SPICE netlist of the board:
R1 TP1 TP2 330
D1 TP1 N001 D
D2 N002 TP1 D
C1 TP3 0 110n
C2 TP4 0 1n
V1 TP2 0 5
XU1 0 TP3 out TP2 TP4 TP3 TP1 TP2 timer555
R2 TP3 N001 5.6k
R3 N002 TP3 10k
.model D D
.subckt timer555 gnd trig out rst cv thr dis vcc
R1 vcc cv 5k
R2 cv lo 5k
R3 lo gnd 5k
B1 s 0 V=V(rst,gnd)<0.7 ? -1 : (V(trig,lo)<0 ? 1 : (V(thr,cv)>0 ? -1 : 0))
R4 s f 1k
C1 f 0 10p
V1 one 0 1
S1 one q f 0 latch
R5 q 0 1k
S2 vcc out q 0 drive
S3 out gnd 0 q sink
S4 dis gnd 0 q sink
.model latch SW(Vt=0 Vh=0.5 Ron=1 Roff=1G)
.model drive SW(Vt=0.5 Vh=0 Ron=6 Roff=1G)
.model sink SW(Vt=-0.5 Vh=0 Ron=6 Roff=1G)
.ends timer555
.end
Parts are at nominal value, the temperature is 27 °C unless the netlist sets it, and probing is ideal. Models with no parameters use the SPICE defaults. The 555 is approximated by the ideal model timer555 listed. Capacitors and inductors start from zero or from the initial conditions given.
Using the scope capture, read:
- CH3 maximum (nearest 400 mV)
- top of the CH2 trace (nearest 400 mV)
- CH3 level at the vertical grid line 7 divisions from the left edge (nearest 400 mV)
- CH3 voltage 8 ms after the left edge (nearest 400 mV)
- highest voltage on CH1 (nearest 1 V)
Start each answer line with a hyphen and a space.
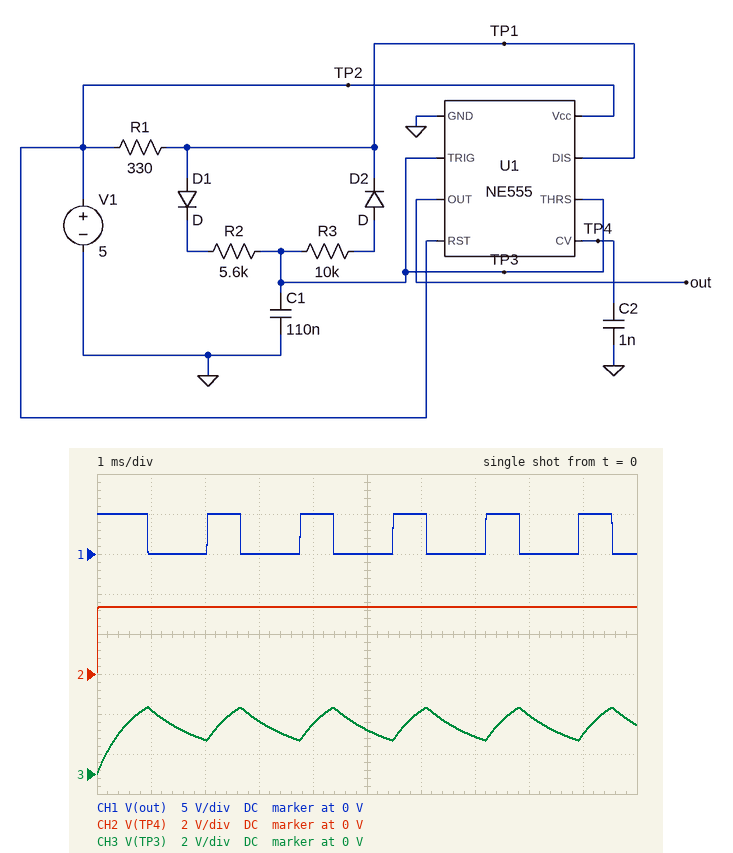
- 3.2 V
- 3.2 V
- 2.0 V
- 2.8 V
- 5 V
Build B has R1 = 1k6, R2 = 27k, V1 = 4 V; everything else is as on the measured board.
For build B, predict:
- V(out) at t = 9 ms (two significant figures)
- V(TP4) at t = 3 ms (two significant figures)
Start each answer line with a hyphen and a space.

- 4.0 V
- 2.7 V
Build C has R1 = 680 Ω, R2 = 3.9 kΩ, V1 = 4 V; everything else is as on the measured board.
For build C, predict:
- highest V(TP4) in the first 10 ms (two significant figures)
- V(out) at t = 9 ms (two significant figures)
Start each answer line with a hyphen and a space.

- 2.7 V
- 4.0 V
